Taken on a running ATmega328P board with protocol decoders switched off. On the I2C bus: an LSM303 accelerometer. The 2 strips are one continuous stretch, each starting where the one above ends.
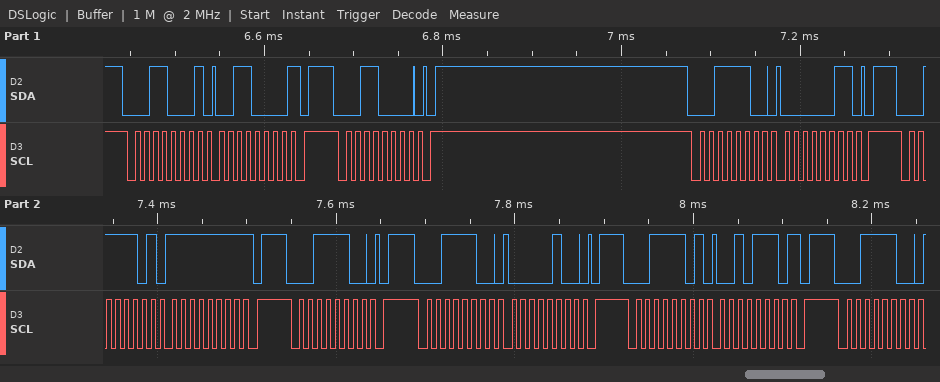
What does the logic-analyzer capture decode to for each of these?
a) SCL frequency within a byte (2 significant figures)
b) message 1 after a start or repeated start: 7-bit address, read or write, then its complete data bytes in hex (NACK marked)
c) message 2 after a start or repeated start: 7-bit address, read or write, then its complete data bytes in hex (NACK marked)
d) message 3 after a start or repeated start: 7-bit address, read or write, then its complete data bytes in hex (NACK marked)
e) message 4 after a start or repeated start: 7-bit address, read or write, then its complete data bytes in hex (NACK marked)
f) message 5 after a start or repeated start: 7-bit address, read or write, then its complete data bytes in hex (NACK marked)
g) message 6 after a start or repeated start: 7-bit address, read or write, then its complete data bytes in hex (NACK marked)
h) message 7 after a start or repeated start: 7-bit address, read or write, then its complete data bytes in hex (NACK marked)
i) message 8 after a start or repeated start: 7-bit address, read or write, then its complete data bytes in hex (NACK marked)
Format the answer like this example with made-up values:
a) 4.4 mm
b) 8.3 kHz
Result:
a) 100 kHz
b) 0x18 read: 30 NACK
c) 0x18 write
d) 0x1E write: 03
e) 0x1E read: FF NACK
f) 0x1E write
g) 0x1E write: 04
h) 0x1E read: 2E NACK
i) 0x1E write
